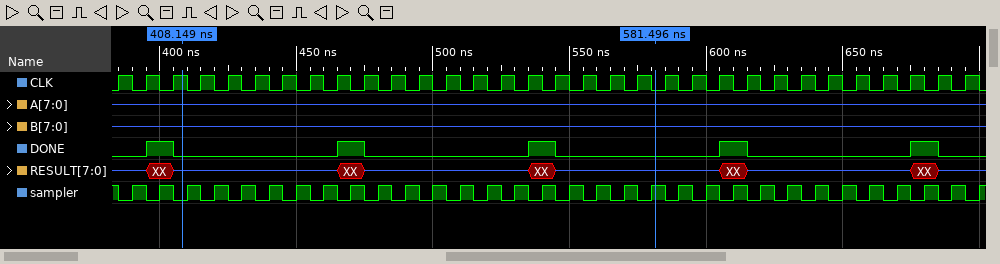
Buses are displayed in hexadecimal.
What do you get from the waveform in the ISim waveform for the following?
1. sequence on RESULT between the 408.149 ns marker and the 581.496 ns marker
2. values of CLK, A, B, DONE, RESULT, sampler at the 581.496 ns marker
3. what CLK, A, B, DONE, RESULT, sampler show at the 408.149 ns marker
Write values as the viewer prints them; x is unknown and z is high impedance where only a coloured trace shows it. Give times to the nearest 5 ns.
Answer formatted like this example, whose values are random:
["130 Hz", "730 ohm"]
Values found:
["z, XX, z, XX, z", "CLK=0, A=z, B=z, DONE=0, RESULT=z, sampler=1", "CLK=1, A=z, B=z, DONE=0, RESULT=z, sampler=0"]
